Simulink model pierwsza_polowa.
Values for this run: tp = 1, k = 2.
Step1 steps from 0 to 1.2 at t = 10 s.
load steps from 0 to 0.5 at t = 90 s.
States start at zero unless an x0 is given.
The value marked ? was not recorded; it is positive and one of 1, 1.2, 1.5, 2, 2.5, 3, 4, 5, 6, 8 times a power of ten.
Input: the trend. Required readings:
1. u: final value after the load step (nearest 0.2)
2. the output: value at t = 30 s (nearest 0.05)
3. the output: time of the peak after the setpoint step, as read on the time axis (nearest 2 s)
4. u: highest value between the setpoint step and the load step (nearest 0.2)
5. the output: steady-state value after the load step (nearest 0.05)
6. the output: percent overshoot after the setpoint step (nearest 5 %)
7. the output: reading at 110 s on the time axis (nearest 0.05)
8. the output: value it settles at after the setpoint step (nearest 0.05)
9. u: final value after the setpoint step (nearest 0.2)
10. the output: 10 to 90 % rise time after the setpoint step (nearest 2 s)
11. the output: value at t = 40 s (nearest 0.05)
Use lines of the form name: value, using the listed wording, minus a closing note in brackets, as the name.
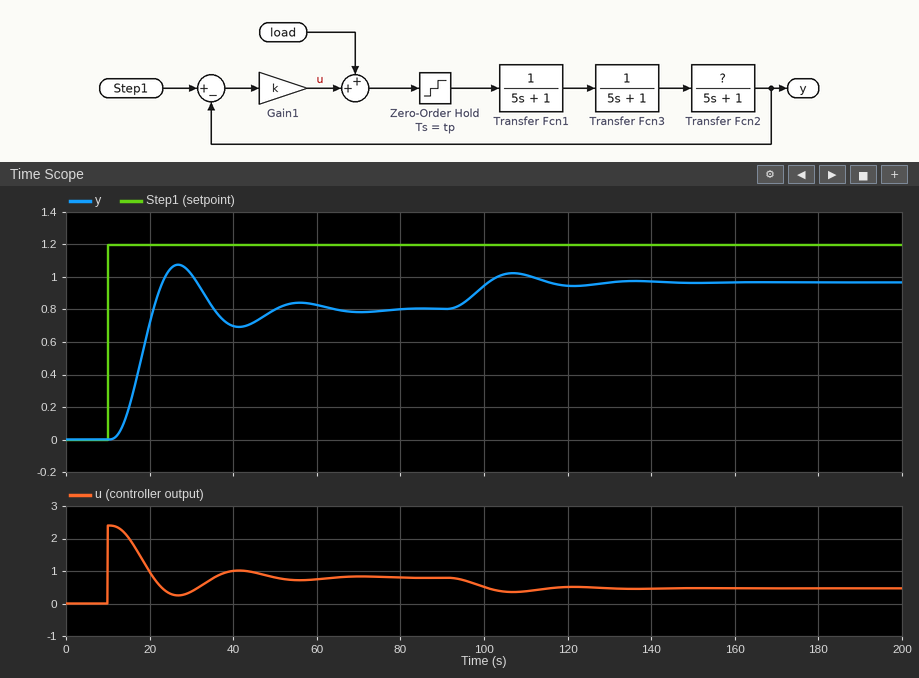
u: final value after the load step: 0.4
the output: value at t = 30 s: 1.00
the output: time of the peak after the setpoint step, as read on the time axis: 26 s
u: highest value between the setpoint step and the load step: 2.4
the output: steady-state value after the load step: 0.95
the output: percent overshoot after the setpoint step: 35 %
the output: reading at 110 s on the time axis: 1.00
the output: value it settles at after the setpoint step: 0.80
u: final value after the setpoint step: 0.8
the output: 10 to 90 % rise time after the setpoint step: 6 s
the output: value at t = 40 s: 0.70
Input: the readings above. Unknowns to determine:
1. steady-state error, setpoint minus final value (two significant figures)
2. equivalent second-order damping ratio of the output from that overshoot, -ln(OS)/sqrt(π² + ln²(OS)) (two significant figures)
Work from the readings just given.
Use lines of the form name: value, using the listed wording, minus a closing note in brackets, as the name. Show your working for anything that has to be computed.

steady-state error, setpoint minus final value: 1.2 - 0.8 = 0.40
equivalent second-order damping ratio of the output from that overshoot, -ln(OS)/sqrt(π² + ln²(OS)): ln(0.35) = -1.050; 1.050 / sqrt(9.870 + 1.102) = 0.32
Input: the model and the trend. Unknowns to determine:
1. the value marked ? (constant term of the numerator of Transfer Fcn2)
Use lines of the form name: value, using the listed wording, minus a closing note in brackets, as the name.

the value marked ?: 1
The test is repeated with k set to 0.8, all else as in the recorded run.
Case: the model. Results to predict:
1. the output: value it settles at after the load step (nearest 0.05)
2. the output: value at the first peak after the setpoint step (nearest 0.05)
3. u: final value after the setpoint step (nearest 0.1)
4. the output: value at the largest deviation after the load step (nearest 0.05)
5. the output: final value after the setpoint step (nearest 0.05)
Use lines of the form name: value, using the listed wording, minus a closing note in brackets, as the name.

the output: value it settles at after the load step: 0.80
the output: value at the first peak after the setpoint step: 0.60
u: final value after the setpoint step: 0.5
the output: value at the largest deviation after the load step: 0.85
the output: final value after the setpoint step: 0.55
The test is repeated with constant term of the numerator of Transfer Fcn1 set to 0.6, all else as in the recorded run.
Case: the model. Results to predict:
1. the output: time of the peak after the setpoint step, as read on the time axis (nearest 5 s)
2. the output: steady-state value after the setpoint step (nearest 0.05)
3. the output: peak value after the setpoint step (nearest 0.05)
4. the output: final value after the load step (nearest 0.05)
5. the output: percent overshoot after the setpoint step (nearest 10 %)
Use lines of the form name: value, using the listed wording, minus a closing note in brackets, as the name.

the output: time of the peak after the setpoint step, as read on the time axis: 30 s
the output: steady-state value after the setpoint step: 0.65
the output: peak value after the setpoint step: 0.80
the output: final value after the load step: 0.80
the output: percent overshoot after the setpoint step: 20 %
